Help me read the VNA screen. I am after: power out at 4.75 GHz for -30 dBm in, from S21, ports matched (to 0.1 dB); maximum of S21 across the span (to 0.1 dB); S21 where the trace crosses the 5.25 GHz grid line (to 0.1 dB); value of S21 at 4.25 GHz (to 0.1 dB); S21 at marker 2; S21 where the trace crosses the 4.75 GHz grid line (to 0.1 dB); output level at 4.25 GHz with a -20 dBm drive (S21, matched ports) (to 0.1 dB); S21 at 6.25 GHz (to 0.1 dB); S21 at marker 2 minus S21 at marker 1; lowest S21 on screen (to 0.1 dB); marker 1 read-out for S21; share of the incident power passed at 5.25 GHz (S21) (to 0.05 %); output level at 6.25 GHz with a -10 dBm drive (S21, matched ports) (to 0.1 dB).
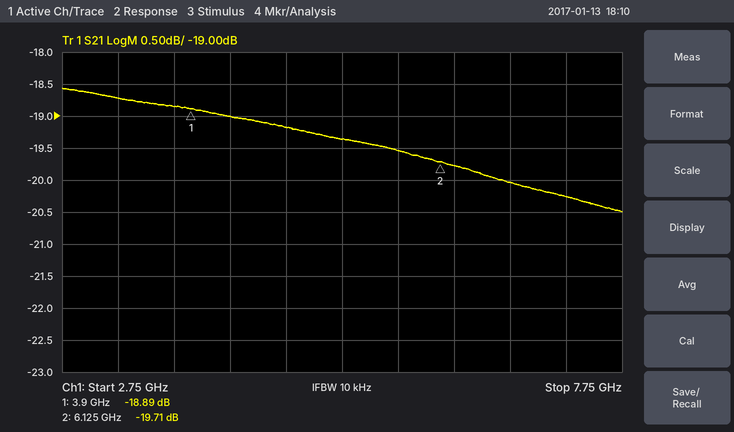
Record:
-49.2 dBm
-18.6 dB
-19.4 dB
-19.0 dB
-19.71 dB
-19.2 dB
-39.0 dBm
-19.8 dB
-0.82 dB
-20.5 dB
-18.89 dB
1.15 %
-29.8 dBm
